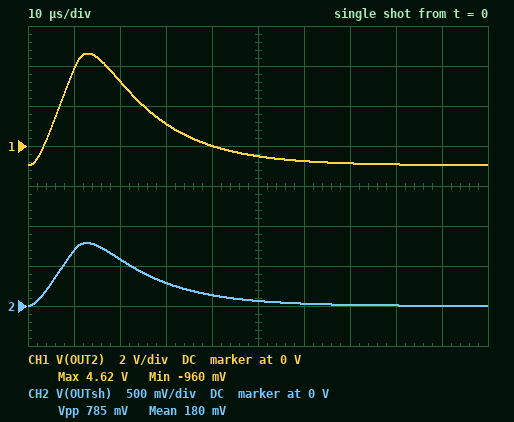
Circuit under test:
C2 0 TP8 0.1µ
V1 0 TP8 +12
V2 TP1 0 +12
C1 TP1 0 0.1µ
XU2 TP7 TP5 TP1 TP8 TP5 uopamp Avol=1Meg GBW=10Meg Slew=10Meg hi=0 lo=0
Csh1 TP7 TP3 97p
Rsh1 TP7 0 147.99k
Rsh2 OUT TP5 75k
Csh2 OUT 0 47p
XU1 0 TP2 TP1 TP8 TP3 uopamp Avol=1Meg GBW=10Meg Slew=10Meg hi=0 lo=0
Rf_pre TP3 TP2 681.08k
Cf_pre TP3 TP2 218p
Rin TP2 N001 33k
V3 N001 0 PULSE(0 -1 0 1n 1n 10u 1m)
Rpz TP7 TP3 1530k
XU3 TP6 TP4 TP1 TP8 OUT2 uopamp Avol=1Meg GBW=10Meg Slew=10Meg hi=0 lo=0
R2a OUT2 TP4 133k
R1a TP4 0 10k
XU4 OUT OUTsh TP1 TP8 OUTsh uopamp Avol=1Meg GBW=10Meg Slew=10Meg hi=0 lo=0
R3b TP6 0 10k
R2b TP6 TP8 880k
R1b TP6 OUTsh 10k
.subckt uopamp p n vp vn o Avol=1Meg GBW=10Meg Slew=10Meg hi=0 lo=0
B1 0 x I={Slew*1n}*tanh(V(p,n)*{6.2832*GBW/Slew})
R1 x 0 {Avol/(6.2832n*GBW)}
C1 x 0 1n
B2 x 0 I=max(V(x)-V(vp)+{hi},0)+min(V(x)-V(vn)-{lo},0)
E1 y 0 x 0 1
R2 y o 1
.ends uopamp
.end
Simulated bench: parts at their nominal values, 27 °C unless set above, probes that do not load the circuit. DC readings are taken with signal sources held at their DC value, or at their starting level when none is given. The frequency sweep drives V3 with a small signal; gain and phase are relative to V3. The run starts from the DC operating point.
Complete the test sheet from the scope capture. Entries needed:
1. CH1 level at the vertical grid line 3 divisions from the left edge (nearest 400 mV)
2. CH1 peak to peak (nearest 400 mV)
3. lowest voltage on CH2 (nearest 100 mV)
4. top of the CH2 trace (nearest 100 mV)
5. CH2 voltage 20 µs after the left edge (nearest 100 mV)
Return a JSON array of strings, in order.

["1.2 V", "5.6 V", "0 V", "800 mV", "600 mV"]
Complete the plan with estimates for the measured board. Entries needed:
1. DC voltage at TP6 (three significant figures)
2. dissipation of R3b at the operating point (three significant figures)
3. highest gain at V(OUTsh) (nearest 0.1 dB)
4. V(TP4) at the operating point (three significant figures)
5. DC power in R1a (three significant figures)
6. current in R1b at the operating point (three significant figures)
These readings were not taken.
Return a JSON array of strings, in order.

["-67.8 mV", "460 nW", "5.2 dB", "-67.8 mV", "460 nW", "6.78 µA"]
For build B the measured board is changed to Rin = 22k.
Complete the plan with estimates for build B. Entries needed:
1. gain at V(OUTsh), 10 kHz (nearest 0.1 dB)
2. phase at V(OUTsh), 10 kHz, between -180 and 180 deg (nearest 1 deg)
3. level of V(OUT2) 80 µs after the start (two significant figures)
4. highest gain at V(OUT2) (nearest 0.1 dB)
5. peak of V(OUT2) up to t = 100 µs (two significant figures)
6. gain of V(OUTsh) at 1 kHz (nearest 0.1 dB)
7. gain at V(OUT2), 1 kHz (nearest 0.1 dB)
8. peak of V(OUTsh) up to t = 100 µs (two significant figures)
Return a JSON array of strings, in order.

["6.2 dB", "128 deg", "-900 mV", "25.8 dB", "7.4 V", "8.7 dB", "25.7 dB", "1.2 V"]
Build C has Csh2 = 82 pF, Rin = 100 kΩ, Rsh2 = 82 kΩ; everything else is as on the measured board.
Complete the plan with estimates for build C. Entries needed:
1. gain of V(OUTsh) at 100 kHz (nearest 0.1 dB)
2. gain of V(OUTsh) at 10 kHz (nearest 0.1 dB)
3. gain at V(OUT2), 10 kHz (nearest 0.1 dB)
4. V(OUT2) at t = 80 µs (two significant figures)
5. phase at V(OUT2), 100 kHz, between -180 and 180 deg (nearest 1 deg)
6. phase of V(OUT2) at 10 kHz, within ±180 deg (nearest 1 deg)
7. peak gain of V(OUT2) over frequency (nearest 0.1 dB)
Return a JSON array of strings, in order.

["-35.6 dB", "-7.4 dB", "9.6 dB", "-950 mV", "10 deg", "117 deg", "12.6 dB"]
